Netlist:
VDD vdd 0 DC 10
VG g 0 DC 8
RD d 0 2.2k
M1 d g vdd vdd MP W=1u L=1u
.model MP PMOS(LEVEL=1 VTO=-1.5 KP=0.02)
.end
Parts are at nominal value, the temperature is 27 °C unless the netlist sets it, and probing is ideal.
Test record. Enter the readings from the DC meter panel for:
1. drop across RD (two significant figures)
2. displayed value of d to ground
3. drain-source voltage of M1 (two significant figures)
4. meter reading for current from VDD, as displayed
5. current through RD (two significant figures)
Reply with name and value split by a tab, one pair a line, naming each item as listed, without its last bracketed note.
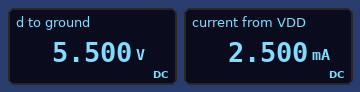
drop across RD	5.5 V
displayed value of d to ground	5.500 V
drain-source voltage of M1	-4.5 V
meter reading for current from VDD, as displayed	2.500 mA
current through RD	2.5 mA
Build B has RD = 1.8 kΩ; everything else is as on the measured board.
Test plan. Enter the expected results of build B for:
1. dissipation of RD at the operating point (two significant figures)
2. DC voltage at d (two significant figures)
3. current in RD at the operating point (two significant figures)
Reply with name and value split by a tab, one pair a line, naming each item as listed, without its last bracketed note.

dissipation of RD at the operating point	11 mW
DC voltage at d	4.5 V
current in RD at the operating point	2.5 mA
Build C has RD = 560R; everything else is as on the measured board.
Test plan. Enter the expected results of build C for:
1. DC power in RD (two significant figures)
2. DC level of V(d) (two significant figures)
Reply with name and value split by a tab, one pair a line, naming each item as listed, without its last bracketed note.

DC power in RD	3.5 mW
DC level of V(d)	1.4 V
